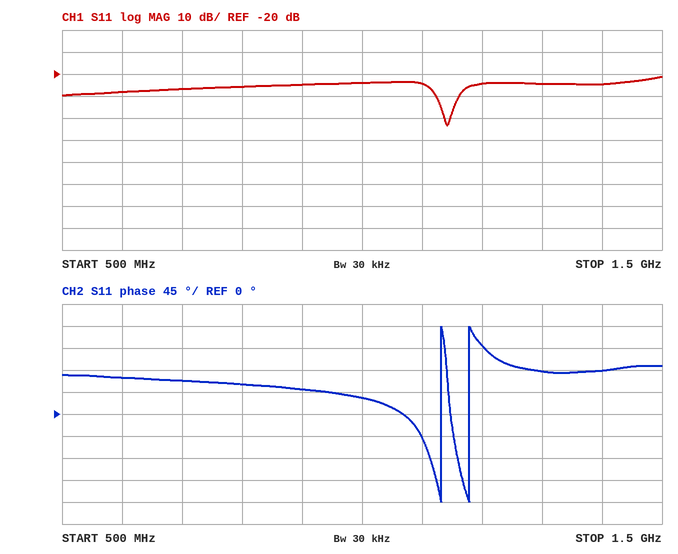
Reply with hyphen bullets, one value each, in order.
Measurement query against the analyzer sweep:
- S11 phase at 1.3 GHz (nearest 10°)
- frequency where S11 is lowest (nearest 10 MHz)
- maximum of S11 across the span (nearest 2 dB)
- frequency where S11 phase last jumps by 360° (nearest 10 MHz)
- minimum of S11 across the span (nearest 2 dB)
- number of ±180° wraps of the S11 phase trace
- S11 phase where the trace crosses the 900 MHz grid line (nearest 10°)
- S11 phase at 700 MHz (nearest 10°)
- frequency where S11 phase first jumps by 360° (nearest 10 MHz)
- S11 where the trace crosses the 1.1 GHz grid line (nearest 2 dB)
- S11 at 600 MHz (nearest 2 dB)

- 90°
- 1.14 GHz
- -22 dB
- 1.18 GHz
- -44 dB
- 2
- 50°
- 70°
- 1.13 GHz
- -24 dB
- -28 dB
